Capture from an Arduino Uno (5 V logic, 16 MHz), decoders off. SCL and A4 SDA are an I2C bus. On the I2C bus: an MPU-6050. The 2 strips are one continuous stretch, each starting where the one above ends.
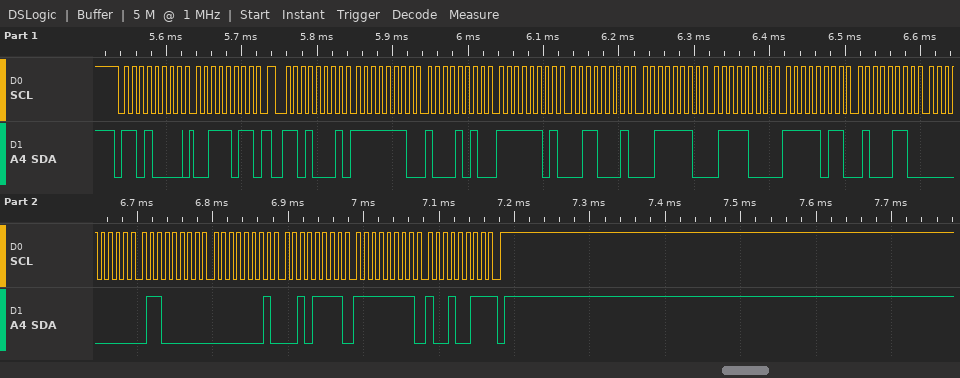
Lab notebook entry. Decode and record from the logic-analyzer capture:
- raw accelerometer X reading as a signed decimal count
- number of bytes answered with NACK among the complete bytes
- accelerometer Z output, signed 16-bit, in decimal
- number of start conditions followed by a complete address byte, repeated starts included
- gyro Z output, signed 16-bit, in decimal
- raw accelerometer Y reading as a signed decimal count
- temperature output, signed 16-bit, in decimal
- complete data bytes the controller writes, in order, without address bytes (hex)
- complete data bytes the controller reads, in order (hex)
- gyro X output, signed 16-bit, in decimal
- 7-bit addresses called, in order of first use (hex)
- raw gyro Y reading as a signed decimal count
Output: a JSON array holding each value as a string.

["-374", "1", "15992", "2", "-109", "-719", "-1210", "3B", "FE 8A FD 31 3E 78 FB 46 00 60 01 2F FF 93", "96", "0x68", "303"]
